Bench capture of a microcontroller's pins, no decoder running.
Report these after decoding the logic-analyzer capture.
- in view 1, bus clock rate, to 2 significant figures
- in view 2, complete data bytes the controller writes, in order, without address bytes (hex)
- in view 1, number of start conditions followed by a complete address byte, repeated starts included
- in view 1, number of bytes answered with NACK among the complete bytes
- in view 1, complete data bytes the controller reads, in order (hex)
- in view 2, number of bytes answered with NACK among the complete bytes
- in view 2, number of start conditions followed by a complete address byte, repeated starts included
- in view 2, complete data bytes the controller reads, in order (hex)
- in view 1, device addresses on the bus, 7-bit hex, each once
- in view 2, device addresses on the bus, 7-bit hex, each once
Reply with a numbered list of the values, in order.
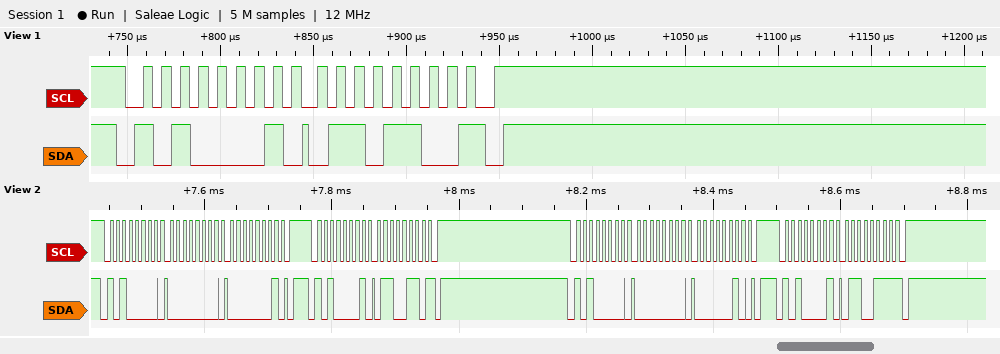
1. 100 kHz
2. 00 01 00 02
3. 1
4. 1
5. 6C
6. 2
7. 4
8. 66 67
9. 0x50
10. 0x50
